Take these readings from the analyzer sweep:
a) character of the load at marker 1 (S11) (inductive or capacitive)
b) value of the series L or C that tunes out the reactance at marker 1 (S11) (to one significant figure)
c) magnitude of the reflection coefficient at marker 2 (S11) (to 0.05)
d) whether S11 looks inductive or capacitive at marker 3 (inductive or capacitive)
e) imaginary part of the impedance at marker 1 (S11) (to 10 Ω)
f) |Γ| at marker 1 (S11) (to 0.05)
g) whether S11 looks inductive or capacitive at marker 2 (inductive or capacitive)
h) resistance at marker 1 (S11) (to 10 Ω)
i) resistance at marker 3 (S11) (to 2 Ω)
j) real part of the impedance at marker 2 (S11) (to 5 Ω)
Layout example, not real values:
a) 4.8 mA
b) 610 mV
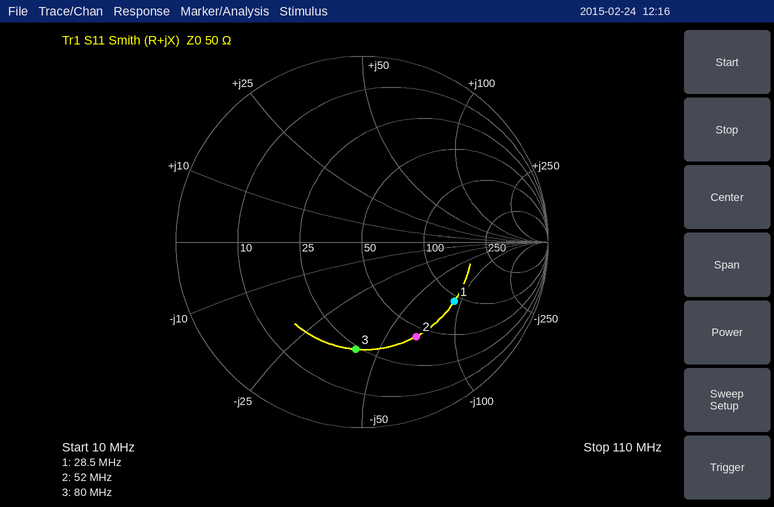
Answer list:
a) capacitive
b) 500 nH
c) 0.60
d) capacitive
e) -90 Ω
f) 0.60
g) capacitive
h) 90 Ω
i) 24 Ω
j) 45 Ω
